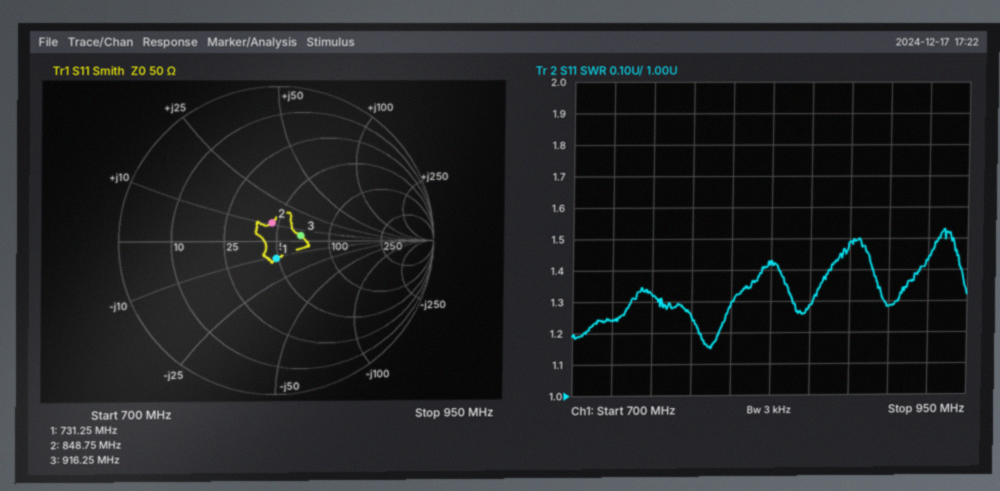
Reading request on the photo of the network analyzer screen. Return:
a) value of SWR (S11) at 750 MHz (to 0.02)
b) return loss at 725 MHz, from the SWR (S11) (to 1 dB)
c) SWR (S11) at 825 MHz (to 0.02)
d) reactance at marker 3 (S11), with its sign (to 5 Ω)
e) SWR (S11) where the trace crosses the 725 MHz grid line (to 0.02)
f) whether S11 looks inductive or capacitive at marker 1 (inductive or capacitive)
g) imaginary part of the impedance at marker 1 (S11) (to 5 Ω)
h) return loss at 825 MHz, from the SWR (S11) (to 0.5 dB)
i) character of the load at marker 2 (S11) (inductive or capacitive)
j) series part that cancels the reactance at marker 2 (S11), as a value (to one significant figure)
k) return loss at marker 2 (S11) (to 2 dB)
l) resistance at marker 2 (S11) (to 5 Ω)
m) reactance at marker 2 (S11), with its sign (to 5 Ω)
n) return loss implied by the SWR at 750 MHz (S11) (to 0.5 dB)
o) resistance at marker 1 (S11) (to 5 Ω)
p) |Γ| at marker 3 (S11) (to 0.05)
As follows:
1.32
19 dB
1.42
+5 Ω
1.24
capacitive
-10 Ω
15.0 dB
inductive
20 pF
18 dB
45 Ω
+10 Ω
17.0 dB
50 Ω
0.15
